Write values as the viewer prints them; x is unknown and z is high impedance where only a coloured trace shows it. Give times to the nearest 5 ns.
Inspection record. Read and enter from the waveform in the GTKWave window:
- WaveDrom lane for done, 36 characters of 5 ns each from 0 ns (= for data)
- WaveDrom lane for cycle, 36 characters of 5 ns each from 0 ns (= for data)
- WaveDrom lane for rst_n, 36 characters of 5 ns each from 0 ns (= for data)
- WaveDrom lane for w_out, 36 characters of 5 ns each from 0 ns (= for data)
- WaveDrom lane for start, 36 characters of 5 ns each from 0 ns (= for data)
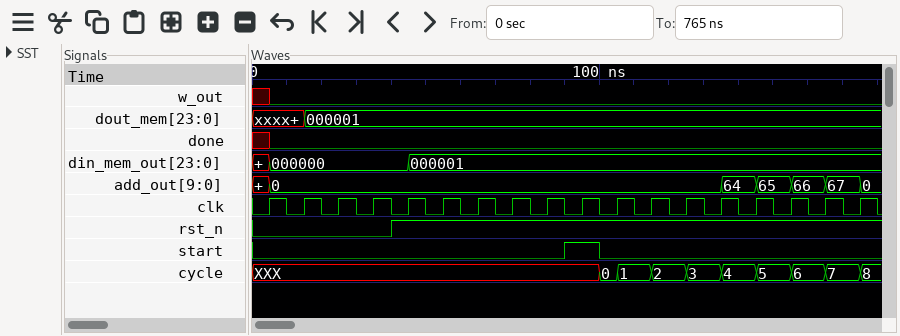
{name: 'done', wave: 'x0..................................'}
{name: 'cycle', wave: 'x...................==.=.=.=.=.=.=.=', data: '0 1 2 3 4 5 6 7 8'}
{name: 'rst_n', wave: '0.......1...........................'}
{name: 'w_out', wave: 'x0..................................'}
{name: 'start', wave: '0.................1.0...............'}
